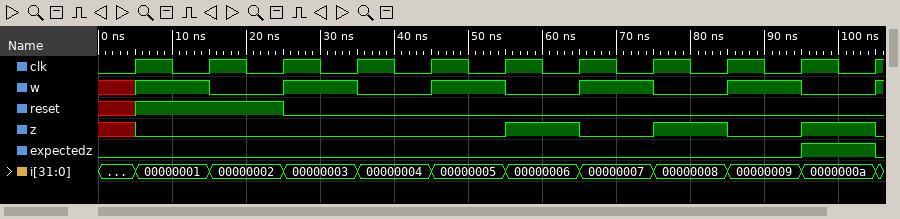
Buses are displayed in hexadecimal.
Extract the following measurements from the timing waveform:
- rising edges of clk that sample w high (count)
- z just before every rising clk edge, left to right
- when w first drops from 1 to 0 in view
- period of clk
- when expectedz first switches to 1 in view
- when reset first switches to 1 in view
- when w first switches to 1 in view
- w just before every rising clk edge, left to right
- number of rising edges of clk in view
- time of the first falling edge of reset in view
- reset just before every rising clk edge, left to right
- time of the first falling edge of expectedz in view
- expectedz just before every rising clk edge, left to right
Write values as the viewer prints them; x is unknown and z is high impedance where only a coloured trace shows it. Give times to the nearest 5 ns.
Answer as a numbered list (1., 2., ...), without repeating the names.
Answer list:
1. 5
2. x 0 0 0 0 0 1 0 1 0 1
3. 15 ns
4. 10 ns
5. 95 ns
6. 5 ns
7. 5 ns
8. x 1 0 1 0 1 0 1 0 1 0
9. 11
10. 25 ns
11. x 1 1 0 0 0 0 0 0 0 0
12. 105 ns
13. 0 0 0 0 0 0 0 0 0 0 1
